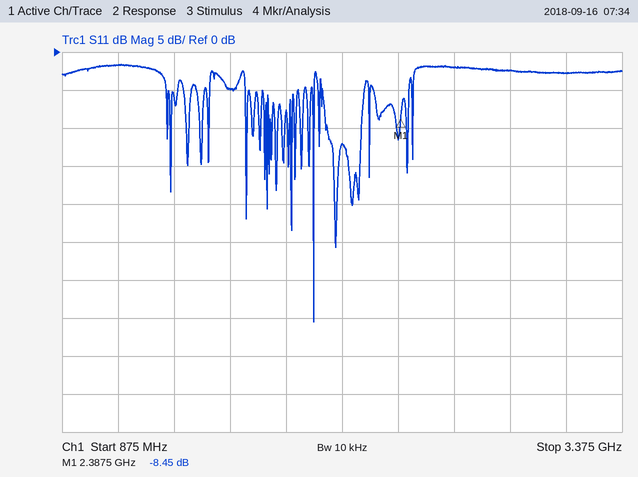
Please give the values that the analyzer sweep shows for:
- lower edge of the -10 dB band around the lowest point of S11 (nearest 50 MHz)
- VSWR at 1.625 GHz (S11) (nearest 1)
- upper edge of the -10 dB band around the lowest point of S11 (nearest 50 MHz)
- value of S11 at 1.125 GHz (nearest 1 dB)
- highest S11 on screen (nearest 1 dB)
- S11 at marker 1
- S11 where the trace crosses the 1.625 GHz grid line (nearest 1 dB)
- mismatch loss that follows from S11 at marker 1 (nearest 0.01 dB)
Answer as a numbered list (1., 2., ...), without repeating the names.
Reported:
1. 2.00 GHz
2. 4
3. 2.00 GHz
4. -2 dB
5. -2 dB
6. -8.45 dB
7. -5 dB
8. 0.67 dB
